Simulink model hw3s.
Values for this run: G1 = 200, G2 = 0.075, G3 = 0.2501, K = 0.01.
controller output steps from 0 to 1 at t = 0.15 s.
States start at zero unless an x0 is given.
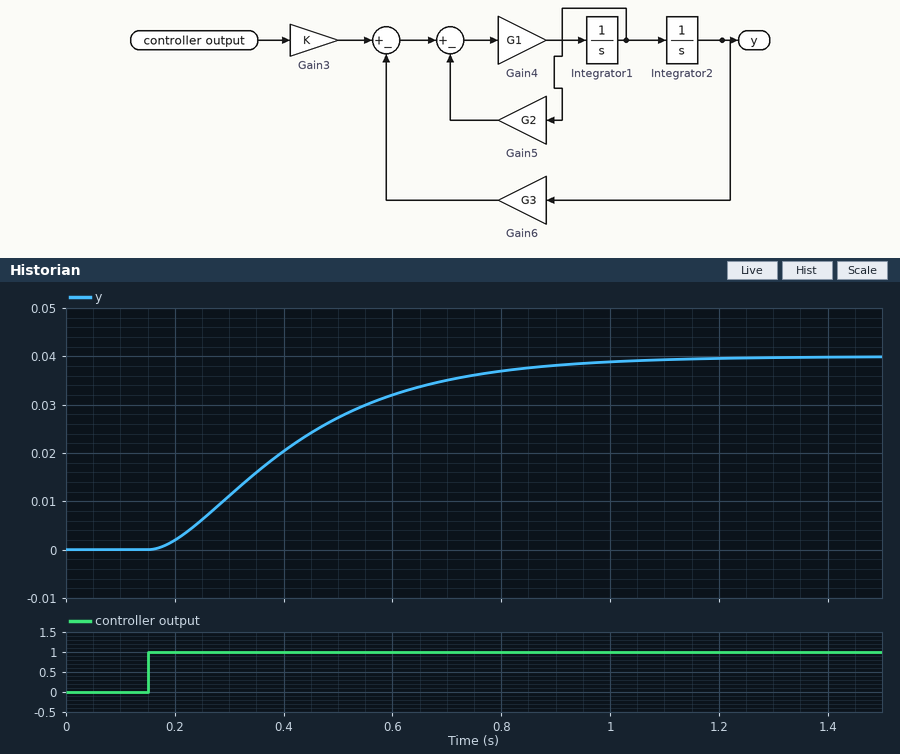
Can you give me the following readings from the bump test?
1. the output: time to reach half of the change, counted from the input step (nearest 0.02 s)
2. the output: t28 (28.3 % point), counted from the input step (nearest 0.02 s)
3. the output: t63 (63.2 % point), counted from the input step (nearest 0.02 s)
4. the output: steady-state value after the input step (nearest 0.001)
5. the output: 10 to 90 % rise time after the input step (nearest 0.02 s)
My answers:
0.24 s
0.16 s
0.32 s
0.040
0.52 s
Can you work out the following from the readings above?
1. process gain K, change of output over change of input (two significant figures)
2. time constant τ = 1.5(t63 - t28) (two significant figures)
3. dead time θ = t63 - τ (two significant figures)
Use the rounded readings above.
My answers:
0.040
0.24 s
0.080 s
